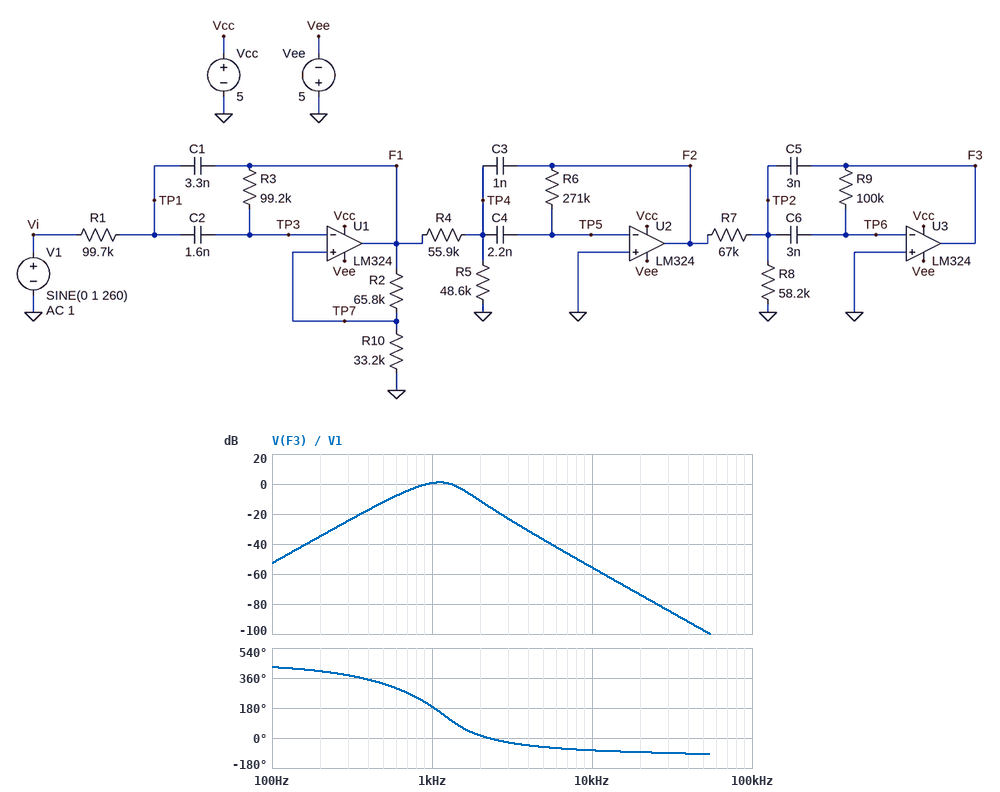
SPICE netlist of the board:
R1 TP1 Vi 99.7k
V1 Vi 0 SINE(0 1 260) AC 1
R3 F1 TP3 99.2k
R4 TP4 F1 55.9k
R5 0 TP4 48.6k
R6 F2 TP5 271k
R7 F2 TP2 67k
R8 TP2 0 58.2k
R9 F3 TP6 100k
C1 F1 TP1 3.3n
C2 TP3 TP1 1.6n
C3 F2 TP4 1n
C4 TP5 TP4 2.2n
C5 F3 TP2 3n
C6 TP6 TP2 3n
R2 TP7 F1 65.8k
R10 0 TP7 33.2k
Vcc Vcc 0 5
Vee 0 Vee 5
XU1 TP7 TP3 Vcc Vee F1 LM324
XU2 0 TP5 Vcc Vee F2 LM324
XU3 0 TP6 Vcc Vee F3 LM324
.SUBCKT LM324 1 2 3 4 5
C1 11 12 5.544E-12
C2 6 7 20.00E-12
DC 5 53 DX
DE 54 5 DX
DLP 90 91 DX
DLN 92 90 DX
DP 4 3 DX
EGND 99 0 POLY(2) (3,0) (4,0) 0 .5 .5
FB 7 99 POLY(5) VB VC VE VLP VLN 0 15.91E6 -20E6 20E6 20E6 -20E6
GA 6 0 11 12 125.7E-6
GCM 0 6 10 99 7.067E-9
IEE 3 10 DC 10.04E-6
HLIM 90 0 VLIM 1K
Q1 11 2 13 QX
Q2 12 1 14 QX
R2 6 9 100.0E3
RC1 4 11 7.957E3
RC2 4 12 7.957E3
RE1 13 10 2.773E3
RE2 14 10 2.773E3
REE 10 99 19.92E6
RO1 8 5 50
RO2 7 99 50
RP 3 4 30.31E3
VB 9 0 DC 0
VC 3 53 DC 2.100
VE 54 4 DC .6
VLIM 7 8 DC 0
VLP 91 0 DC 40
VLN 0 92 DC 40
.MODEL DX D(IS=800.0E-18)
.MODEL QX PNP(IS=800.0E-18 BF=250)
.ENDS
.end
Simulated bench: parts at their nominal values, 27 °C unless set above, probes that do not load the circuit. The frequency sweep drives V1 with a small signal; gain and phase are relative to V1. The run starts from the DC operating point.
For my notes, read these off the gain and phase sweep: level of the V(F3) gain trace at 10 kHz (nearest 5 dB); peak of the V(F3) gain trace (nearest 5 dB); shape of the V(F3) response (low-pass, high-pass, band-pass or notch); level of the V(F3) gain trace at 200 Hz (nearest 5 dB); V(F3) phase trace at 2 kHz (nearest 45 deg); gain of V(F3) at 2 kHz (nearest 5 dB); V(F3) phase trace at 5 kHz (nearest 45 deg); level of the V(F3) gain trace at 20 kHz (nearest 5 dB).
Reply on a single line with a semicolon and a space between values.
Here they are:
-55 dB; 0 dB; band-pass; -35 dB; 0 deg; -10 dB; -45 deg; -75 dB
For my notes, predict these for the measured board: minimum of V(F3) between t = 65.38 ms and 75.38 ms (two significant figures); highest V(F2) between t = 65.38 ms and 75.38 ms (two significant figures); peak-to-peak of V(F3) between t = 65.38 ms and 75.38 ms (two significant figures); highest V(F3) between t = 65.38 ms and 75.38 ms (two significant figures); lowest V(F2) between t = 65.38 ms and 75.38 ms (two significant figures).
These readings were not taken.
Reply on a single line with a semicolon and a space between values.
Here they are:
-41 mV; 160 mV; 78 mV; 37 mV; -170 mV
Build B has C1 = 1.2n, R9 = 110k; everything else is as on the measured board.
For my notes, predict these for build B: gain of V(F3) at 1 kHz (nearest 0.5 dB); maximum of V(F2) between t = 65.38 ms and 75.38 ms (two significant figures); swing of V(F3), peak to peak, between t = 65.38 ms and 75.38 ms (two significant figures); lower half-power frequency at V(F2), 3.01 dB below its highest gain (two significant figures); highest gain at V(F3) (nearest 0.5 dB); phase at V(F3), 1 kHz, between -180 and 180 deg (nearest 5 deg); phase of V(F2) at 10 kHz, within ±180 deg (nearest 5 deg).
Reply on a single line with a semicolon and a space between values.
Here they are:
8.0 dB; 180 mV; 94 mV; 940 Hz; 9.0 dB; -145 deg; -165 deg
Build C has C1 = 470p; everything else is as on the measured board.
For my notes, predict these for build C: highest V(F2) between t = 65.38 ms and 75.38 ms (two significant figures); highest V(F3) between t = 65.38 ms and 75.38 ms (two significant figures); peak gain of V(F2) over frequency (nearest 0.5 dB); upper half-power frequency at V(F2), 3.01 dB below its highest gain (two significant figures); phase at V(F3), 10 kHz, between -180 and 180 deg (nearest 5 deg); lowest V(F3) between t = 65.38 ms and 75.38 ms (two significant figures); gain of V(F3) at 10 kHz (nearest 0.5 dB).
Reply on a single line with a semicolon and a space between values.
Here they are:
180 mV; 41 mV; 15.0 dB; 1.9 kHz; -65 deg; -45 mV; -39.0 dB
